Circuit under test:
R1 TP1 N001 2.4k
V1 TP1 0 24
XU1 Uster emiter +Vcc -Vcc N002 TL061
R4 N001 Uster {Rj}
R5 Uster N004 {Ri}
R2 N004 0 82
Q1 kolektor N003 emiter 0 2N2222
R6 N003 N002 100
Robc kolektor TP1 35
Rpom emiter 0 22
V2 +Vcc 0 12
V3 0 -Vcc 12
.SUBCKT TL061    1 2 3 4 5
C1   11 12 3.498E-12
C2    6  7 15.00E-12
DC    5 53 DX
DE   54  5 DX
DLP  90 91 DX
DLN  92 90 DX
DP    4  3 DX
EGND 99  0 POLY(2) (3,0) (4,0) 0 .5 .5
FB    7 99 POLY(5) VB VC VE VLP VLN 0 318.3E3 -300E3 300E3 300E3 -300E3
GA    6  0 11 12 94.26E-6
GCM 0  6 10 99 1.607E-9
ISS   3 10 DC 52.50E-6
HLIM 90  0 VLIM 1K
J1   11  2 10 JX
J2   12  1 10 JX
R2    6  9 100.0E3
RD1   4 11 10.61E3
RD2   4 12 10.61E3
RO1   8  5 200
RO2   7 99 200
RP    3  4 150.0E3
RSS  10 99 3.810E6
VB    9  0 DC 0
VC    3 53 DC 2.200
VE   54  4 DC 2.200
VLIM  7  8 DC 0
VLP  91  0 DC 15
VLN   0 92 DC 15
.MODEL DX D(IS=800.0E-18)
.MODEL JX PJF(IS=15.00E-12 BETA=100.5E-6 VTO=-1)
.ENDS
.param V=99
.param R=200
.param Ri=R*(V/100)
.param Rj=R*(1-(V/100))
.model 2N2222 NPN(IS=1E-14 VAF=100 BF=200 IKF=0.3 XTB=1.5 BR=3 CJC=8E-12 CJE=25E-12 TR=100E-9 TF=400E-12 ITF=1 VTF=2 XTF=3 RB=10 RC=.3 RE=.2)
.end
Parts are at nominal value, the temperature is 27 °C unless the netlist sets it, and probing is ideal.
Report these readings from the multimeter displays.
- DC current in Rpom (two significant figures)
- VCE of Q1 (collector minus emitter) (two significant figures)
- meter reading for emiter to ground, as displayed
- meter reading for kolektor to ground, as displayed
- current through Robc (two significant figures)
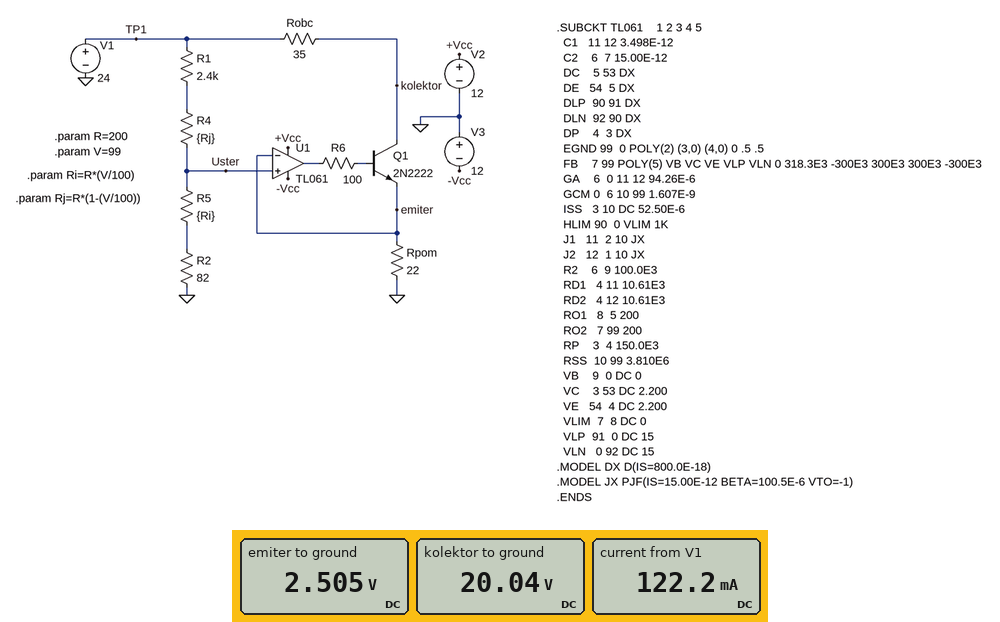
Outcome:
110 mA
18 V
2.505 V
20.04 V
110 mA
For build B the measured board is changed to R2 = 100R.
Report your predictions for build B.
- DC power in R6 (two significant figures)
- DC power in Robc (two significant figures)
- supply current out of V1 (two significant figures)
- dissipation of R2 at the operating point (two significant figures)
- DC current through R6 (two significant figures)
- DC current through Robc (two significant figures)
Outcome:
48 µW
500 mW
130 mA
7.9 mW
690 µA
120 mA
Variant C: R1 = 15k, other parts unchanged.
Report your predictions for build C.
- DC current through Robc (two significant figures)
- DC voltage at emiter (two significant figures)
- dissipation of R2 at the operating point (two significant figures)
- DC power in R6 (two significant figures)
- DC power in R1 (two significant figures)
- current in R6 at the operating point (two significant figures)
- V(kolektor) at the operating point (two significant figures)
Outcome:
20 mA
440 mV
200 µW
740 nW
37 mW
86 µA
23 V
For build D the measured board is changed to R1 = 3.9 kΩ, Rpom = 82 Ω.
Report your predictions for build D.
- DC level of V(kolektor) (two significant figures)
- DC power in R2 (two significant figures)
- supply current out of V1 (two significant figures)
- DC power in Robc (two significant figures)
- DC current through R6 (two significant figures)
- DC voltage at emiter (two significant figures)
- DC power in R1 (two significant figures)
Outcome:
23 V
2.7 mW
25 mA
13 mW
85 µA
1.6 V
130 mW
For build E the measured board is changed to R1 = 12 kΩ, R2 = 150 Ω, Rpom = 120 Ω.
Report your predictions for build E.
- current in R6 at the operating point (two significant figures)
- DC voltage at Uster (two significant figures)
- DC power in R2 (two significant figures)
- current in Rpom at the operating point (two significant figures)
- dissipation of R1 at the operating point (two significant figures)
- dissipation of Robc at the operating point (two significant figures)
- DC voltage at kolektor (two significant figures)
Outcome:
23 µA
680 mV
570 µW
5.6 mA
45 mW
1.1 mW
24 V
